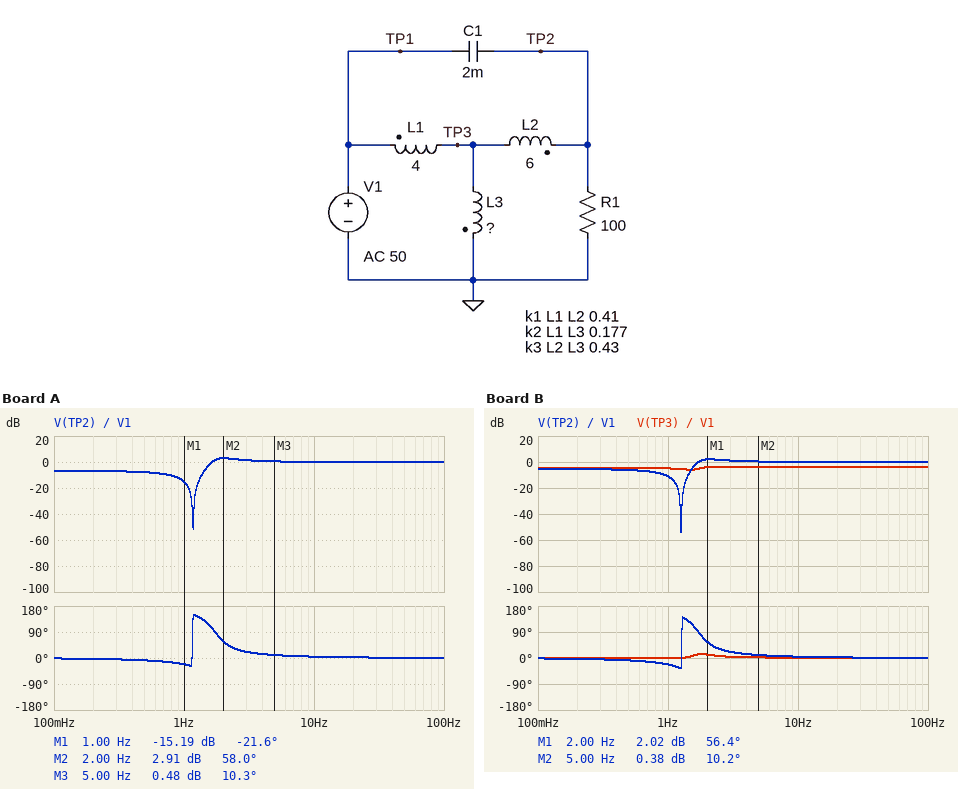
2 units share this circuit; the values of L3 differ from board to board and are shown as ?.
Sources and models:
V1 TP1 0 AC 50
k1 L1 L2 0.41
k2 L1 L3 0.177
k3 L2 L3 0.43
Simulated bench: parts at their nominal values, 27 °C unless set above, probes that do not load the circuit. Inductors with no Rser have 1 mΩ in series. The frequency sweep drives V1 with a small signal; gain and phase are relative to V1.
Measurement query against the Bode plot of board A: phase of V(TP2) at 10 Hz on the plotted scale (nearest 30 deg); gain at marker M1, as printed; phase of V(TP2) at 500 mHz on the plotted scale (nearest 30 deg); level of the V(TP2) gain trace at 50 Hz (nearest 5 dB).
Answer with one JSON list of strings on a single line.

["0 deg", "-15.19 dB", "0 deg", "0 dB"]
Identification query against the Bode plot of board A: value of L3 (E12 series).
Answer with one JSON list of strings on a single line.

["3.3 H"]
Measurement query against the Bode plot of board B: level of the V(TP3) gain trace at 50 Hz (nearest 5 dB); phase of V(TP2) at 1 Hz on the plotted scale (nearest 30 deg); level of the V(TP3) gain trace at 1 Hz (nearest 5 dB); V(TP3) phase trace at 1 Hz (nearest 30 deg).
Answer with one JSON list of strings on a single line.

["-5 dB", "-30 deg", "-5 dB", "0 deg"]
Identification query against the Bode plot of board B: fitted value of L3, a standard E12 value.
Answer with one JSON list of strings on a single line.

["5.6 H"]
